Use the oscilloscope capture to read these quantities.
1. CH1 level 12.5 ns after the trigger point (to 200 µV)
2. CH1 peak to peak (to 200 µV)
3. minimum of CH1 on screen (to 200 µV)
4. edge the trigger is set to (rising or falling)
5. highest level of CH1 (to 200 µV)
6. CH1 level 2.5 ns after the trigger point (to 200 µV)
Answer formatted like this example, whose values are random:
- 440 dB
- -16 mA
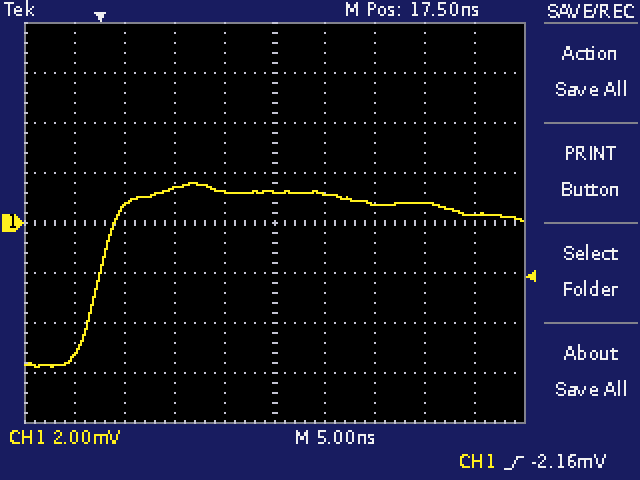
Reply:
- 1.2 mV
- 7.4 mV
- -5.8 mV
- rising
- 1.6 mV
- 600 µV
